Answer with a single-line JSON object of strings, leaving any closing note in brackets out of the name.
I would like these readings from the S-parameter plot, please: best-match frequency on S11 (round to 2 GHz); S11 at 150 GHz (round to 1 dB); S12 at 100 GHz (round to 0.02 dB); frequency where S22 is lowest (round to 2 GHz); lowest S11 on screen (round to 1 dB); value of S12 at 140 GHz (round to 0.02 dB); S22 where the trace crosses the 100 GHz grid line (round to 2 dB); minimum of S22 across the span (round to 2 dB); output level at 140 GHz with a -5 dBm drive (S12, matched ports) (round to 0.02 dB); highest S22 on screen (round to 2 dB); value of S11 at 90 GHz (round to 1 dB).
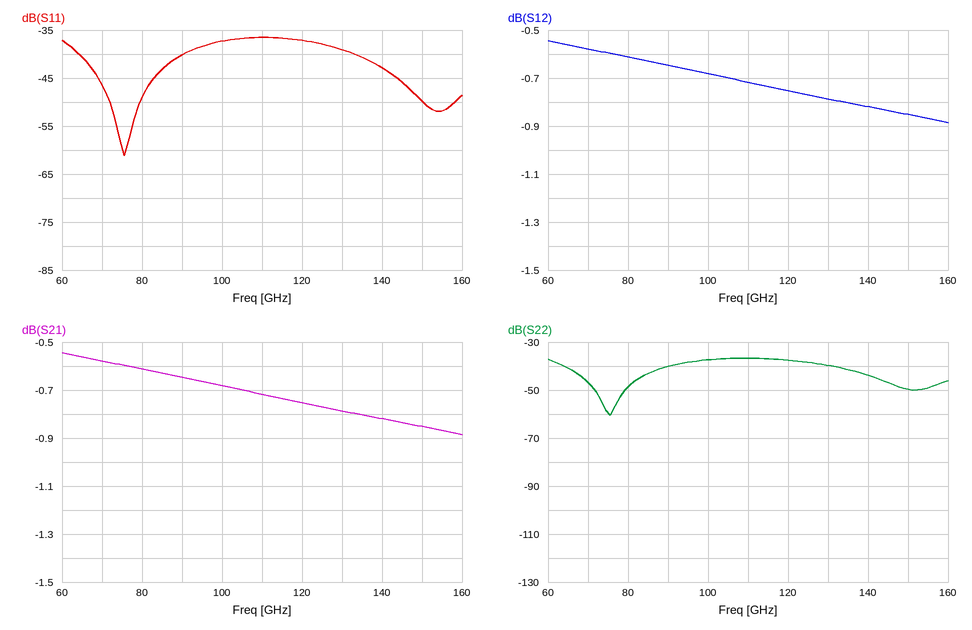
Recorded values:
{"best-match frequency on S11": "76 GHz", "S11 at 150 GHz": "-50 dB", "S12 at 100 GHz": "-0.68 dB", "frequency where S22 is lowest": "76 GHz", "lowest S11 on screen": "-61 dB", "value of S12 at 140 GHz": "-0.82 dB", "S22 where the trace crosses the 100 GHz grid line": "-38 dB", "minimum of S22 across the span": "-60 dB", "output level at 140 GHz with a -5 dBm drive (S12, matched ports)": "-5.82 dBm", "highest S22 on screen": "-36 dB", "value of S11 at 90 GHz": "-40 dB"}
